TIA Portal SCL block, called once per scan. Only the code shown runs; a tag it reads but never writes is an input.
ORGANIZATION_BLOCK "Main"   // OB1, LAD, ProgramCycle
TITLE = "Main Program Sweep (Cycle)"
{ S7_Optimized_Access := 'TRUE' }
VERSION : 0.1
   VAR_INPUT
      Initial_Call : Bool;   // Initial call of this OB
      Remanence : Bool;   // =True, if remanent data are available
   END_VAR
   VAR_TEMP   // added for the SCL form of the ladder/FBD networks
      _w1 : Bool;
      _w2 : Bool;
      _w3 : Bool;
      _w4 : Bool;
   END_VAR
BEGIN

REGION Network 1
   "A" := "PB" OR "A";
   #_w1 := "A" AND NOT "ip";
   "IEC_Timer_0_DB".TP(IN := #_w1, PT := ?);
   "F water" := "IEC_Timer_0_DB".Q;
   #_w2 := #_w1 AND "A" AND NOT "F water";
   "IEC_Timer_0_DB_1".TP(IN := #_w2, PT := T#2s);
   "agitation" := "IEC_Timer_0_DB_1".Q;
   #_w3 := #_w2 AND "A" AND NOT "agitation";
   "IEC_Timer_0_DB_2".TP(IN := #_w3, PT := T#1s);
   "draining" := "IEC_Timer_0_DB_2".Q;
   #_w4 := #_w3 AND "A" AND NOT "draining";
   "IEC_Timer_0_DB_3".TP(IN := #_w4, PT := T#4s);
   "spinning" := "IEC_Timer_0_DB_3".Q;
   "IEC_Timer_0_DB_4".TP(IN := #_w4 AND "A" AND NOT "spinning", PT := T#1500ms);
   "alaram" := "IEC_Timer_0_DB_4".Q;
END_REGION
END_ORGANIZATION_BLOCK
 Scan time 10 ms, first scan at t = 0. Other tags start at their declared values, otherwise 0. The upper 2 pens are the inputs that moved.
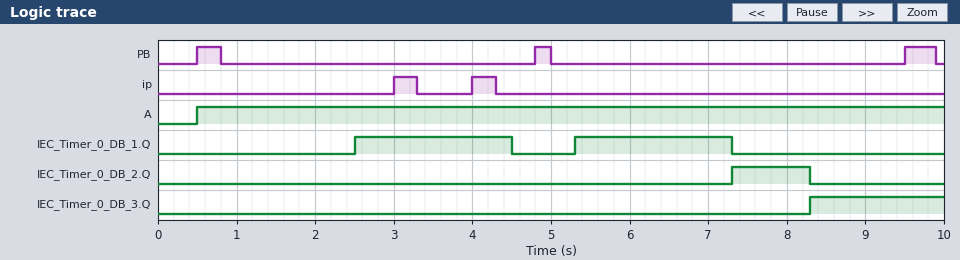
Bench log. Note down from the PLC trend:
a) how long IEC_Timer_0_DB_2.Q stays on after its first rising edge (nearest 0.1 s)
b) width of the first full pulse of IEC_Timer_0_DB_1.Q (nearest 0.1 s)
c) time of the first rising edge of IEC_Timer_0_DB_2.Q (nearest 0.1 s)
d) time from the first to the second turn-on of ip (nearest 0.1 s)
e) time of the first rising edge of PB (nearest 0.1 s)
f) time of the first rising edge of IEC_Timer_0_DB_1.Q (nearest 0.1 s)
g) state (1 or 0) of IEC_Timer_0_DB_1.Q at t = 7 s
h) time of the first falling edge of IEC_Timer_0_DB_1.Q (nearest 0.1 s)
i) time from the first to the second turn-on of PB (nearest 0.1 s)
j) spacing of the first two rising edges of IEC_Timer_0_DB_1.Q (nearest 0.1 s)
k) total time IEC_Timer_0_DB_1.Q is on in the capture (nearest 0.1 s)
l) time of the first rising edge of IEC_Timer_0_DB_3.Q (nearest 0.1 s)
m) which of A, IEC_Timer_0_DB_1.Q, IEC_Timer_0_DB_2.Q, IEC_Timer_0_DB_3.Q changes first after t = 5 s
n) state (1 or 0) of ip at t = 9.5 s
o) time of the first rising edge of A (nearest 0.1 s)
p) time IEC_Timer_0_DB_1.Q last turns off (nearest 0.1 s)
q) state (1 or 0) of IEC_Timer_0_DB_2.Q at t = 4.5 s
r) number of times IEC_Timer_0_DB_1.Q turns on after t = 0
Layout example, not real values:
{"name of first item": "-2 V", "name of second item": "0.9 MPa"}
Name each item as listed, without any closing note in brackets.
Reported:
{"how long IEC_Timer_0_DB_2.Q stays on after its first rising edge": "1.0 s", "width of the first full pulse of IEC_Timer_0_DB_1.Q": "2.0 s", "time of the first rising edge of IEC_Timer_0_DB_2.Q": "7.3 s", "time from the first to the second turn-on of ip": "1.0 s", "time of the first rising edge of PB": "0.5 s", "time of the first rising edge of IEC_Timer_0_DB_1.Q": "2.5 s", "state (1 or 0) of IEC_Timer_0_DB_1.Q at t = 7 s": "1", "time of the first falling edge of IEC_Timer_0_DB_1.Q": "4.5 s", "time from the first to the second turn-on of PB": "4.3 s", "spacing of the first two rising edges of IEC_Timer_0_DB_1.Q": "2.8 s", "total time IEC_Timer_0_DB_1.Q is on in the capture": "4.0 s", "time of the first rising edge of IEC_Timer_0_DB_3.Q": "8.3 s", "which of A, IEC_Timer_0_DB_1.Q, IEC_Timer_0_DB_2.Q, IEC_Timer_0_DB_3.Q changes first after t = 5 s": "IEC_Timer_0_DB_1.Q", "state (1 or 0) of ip at t = 9.5 s": "0", "time of the first rising edge of A": "0.5 s", "time IEC_Timer_0_DB_1.Q last turns off": "7.3 s", "state (1 or 0) of IEC_Timer_0_DB_2.Q at t = 4.5 s": "0", "number of times IEC_Timer_0_DB_1.Q turns on after t = 0": "2"}
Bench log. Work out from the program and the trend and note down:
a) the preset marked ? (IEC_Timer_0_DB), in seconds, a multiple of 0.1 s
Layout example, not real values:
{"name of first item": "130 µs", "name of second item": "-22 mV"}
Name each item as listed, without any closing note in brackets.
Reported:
{"the preset marked ? (IEC_Timer_0_DB), in seconds, a multiple of 0.1 s": "2.0 s"}
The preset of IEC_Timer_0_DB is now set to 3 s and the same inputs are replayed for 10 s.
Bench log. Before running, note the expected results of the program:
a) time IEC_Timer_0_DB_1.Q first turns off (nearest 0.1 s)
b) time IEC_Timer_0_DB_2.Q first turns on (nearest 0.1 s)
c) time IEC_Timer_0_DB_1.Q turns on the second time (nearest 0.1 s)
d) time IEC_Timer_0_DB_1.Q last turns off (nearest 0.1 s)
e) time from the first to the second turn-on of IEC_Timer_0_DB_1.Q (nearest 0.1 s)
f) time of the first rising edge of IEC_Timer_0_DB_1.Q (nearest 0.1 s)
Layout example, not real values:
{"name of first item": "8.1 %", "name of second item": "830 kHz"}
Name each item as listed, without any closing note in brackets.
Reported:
{"time IEC_Timer_0_DB_1.Q first turns off": "5.5 s", "time IEC_Timer_0_DB_2.Q first turns on": "9.3 s", "time IEC_Timer_0_DB_1.Q turns on the second time": "7.3 s", "time IEC_Timer_0_DB_1.Q last turns off": "9.3 s", "time from the first to the second turn-on of IEC_Timer_0_DB_1.Q": "3.8 s", "time of the first rising edge of IEC_Timer_0_DB_1.Q": "3.5 s"}
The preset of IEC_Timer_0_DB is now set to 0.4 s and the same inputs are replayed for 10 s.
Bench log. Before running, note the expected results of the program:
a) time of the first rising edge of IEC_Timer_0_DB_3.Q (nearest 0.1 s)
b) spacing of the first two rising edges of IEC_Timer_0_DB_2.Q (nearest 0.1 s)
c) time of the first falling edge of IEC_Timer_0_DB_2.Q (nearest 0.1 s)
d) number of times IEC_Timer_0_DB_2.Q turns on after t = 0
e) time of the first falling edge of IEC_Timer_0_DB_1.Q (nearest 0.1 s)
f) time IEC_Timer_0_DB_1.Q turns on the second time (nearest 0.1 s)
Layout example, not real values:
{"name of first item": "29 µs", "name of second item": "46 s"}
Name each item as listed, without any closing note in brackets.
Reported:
{"time of the first rising edge of IEC_Timer_0_DB_3.Q": "6.7 s", "spacing of the first two rising edges of IEC_Timer_0_DB_2.Q": "2.8 s", "time of the first falling edge of IEC_Timer_0_DB_2.Q": "3.9 s", "number of times IEC_Timer_0_DB_2.Q turns on after t = 0": "2", "time of the first falling edge of IEC_Timer_0_DB_1.Q": "2.9 s", "time IEC_Timer_0_DB_1.Q turns on the second time": "3.7 s"}
